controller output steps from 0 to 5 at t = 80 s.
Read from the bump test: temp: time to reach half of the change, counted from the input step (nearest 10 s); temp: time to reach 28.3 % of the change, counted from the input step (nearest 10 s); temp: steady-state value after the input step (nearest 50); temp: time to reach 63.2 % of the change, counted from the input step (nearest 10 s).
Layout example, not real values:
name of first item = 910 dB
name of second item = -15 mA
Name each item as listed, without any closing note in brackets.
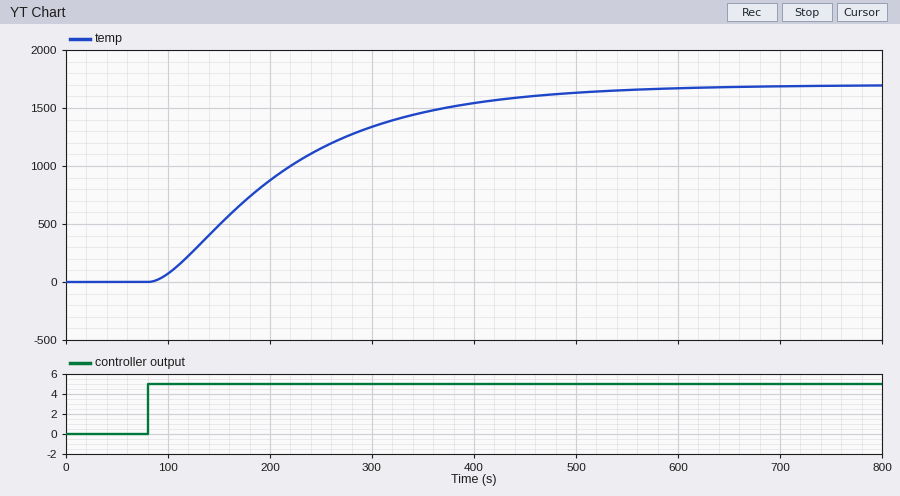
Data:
temp: time to reach half of the change, counted from the input step = 120 s
temp: time to reach 28.3 % of the change, counted from the input step = 70 s
temp: steady-state value after the input step = 1700
temp: time to reach 63.2 % of the change, counted from the input step = 150 s
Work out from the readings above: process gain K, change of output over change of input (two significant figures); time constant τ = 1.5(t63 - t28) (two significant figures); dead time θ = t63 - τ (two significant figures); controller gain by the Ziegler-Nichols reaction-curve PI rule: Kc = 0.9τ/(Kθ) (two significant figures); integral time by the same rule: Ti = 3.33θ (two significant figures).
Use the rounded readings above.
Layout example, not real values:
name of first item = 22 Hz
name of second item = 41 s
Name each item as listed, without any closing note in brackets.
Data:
process gain K, change of output over change of input = 340
time constant τ = 1.5(t63 - t28) = 120 s
dead time θ = t63 - τ = 30 s
controller gain by the Ziegler-Nichols reaction-curve PI rule: Kc = 0.9τ/(Kθ) = 0.011
integral time by the same rule: Ti = 3.33θ = 100 s
